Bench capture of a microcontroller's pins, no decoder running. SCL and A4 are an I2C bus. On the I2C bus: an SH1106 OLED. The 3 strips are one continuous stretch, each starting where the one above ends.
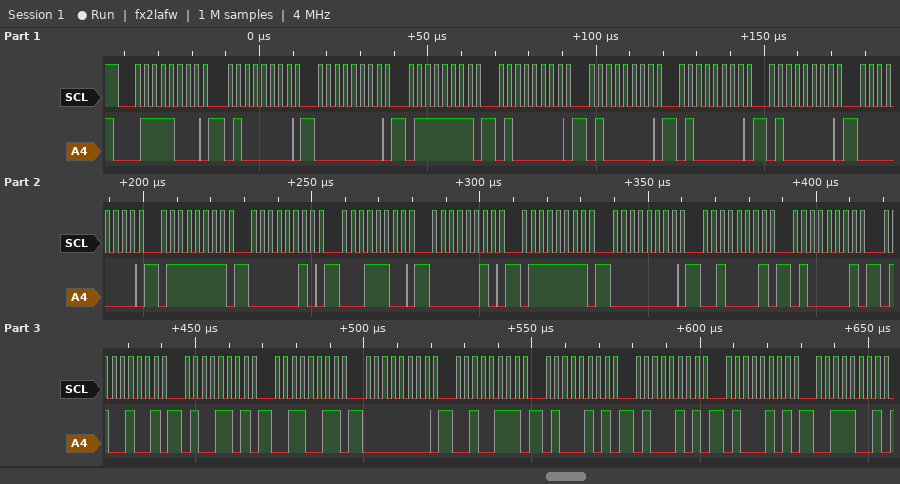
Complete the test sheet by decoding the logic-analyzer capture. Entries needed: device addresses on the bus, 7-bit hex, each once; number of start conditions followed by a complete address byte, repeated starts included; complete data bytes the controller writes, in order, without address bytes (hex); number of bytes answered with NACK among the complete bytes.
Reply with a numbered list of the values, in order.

1. 0x3C
2. 1
3. 40 00 7F 40 40 40 40 00 7F 02 1C 02 7F 00 21 41 49 4D 33 00 27 45 45 45 39
4. 0
